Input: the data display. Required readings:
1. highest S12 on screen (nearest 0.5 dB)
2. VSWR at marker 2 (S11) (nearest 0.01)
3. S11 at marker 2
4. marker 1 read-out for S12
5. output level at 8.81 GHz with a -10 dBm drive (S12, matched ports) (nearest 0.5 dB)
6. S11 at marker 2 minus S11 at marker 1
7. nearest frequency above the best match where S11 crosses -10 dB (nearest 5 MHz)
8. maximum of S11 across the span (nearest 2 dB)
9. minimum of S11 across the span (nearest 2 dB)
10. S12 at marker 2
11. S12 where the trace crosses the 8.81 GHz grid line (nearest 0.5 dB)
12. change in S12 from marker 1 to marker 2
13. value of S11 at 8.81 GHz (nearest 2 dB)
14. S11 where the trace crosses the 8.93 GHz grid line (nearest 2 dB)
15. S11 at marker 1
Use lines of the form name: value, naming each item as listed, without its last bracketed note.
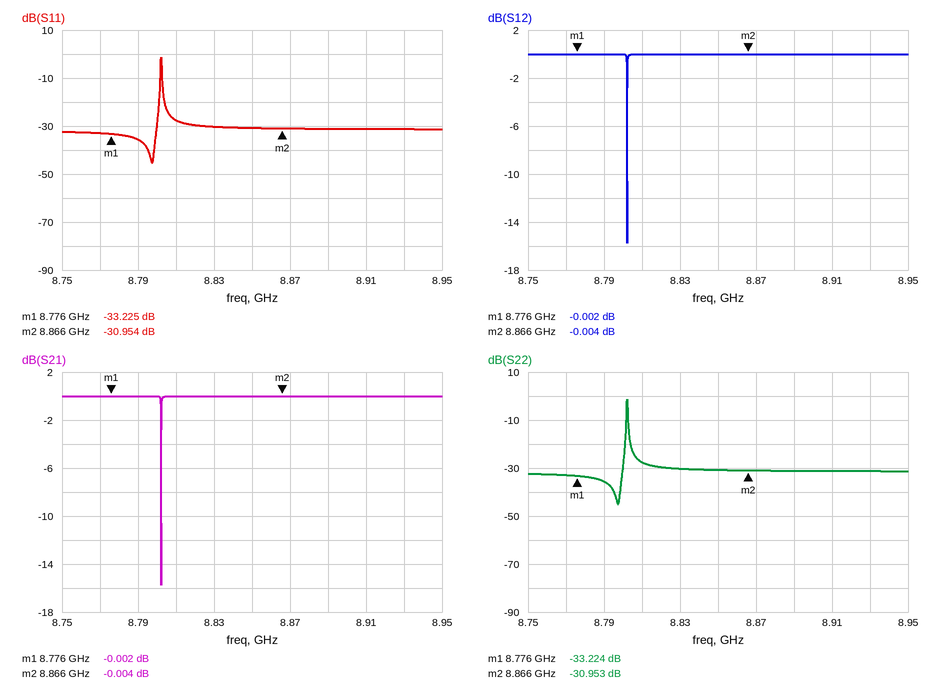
highest S12 on screen: 0.0 dB
VSWR at marker 2 (S11): 1.06
S11 at marker 2: -30.954 dB
marker 1 read-out for S12: -0.002 dB
output level at 8.81 GHz with a -10 dBm drive (S12, matched ports): -10.0 dBm
S11 at marker 2 minus S11 at marker 1: 2.271 dB
nearest frequency above the best match where S11 crosses -10 dB: 8.800 GHz
maximum of S11 across the span: -2 dB
minimum of S11 across the span: -46 dB
S12 at marker 2: -0.004 dB
S12 where the trace crosses the 8.81 GHz grid line: 0.0 dB
change in S12 from marker 1 to marker 2: -0.002 dB
value of S11 at 8.81 GHz: -28 dB
S11 where the trace crosses the 8.93 GHz grid line: -32 dB
S11 at marker 1: -33.225 dB
